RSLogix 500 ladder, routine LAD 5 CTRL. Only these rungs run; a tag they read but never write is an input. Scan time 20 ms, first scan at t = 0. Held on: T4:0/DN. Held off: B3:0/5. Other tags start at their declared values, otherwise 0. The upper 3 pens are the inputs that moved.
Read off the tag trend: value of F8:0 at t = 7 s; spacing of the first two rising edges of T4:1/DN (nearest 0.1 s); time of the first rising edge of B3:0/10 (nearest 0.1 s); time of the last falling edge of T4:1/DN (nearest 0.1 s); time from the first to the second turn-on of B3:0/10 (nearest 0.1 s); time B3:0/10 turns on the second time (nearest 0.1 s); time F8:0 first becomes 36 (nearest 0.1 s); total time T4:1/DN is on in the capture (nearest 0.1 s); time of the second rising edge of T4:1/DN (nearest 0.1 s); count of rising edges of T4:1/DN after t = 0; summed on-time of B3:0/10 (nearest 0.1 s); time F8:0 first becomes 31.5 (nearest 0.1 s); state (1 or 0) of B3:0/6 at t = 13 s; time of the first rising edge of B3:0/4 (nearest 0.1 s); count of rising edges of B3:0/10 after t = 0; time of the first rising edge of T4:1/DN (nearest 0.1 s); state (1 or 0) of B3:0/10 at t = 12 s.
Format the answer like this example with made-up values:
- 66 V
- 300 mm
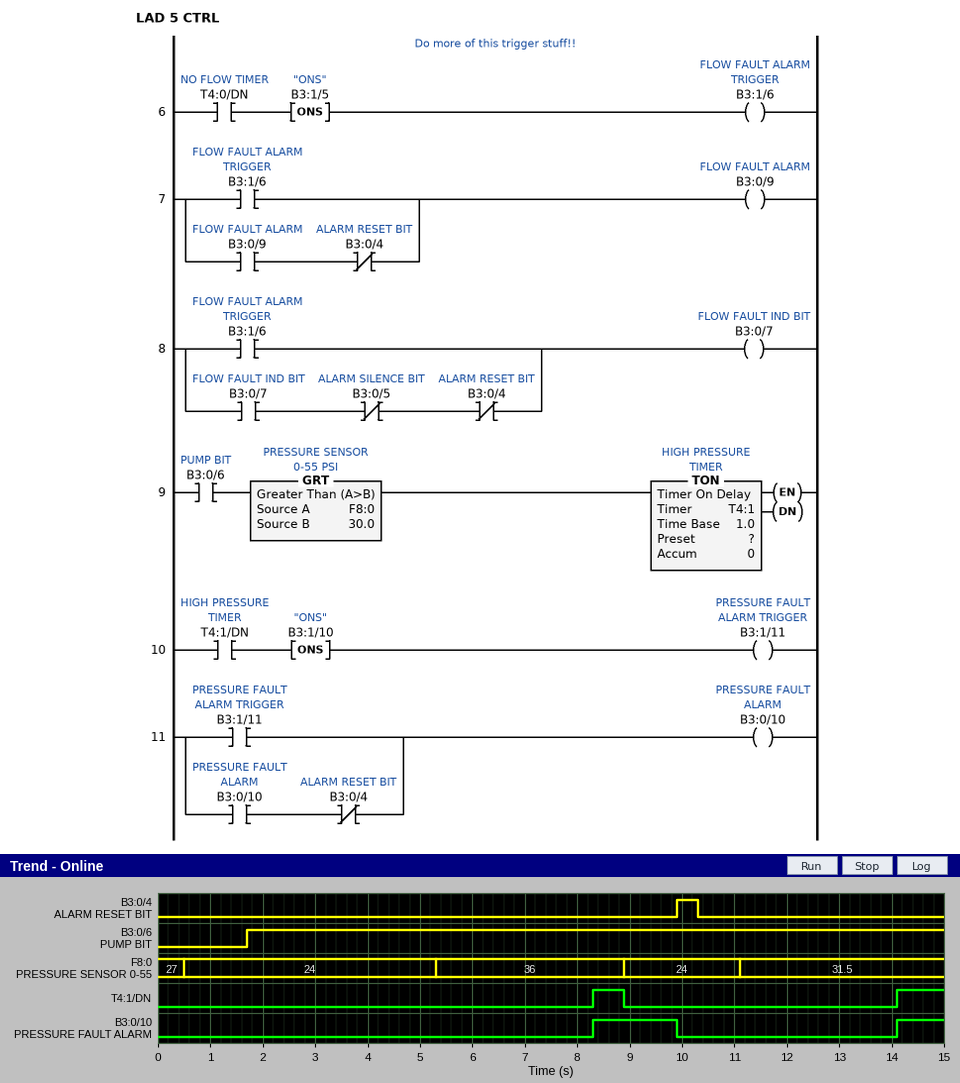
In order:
- 36
- 5.8 s
- 8.3 s
- 8.9 s
- 5.8 s
- 14.1 s
- 5.3 s
- 1.5 s
- 14.1 s
- 2
- 2.5 s
- 11.1 s
- 1
- 9.9 s
- 2
- 8.3 s
- 0
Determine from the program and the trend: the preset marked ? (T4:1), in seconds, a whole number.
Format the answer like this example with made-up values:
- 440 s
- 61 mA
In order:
- 3 s
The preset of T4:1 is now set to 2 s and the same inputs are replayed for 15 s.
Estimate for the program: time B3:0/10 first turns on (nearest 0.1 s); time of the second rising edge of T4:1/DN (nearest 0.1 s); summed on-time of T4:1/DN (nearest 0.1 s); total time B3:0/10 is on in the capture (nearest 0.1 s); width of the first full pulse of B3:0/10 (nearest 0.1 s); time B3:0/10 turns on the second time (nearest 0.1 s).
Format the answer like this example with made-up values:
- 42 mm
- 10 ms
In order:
- 7.3 s
- 13.1 s
- 3.5 s
- 4.5 s
- 2.6 s
- 13.1 s
